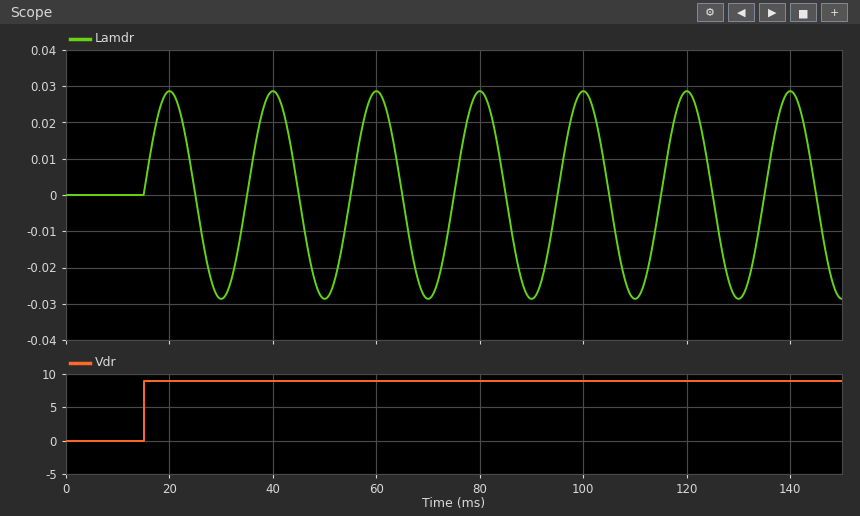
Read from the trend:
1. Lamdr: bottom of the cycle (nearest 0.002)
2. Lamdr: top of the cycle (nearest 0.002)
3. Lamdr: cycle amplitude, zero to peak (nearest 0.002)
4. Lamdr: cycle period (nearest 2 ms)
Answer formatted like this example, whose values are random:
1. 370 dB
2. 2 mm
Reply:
1. -0.028
2. 0.028
3. 0.028
4. 20 ms
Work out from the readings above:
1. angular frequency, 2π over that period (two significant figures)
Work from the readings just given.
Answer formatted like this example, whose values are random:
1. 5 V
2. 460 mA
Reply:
1. 0.31 rad/ms
